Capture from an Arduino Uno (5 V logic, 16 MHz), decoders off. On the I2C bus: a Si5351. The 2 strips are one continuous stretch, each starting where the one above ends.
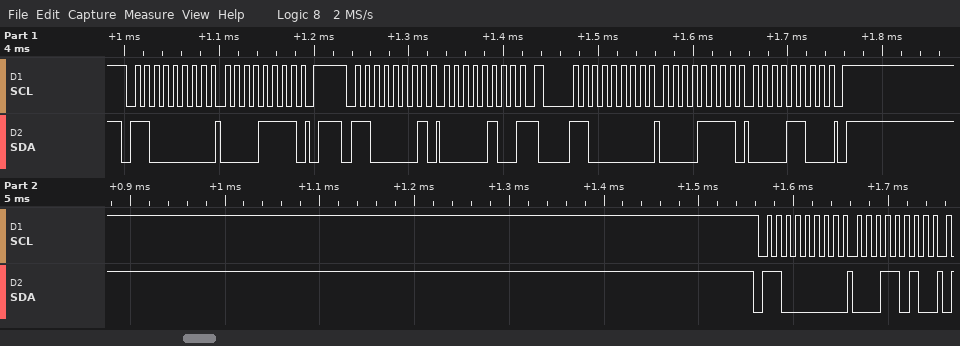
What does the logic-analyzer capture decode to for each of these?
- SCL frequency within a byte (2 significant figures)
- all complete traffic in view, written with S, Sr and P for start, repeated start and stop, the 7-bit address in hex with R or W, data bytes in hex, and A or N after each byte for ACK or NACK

100 kHz
S 60W A 0F A P S 60R A 04 N Sr 60W A 0F A 0C A P S 60W A 1A A
